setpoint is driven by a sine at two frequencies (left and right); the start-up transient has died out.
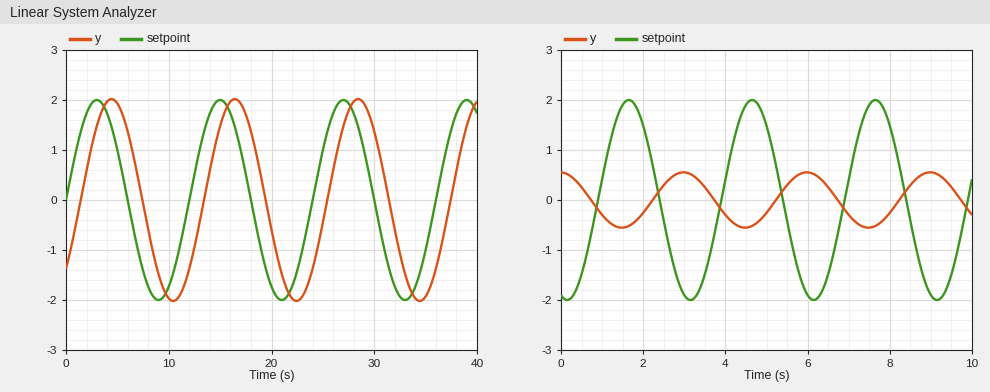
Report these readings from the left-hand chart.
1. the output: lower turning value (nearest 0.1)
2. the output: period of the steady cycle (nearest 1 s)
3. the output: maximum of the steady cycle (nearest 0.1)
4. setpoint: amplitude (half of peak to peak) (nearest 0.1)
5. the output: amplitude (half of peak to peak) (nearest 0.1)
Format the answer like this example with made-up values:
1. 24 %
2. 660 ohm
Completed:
1. -2.0
2. 12 s
3. 2.0
4. 2.0
5. 2.0
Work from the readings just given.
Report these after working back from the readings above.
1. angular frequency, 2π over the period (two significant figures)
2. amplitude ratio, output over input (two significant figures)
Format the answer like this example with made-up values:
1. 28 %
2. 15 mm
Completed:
1. 0.52 rad/s
2. 1.0
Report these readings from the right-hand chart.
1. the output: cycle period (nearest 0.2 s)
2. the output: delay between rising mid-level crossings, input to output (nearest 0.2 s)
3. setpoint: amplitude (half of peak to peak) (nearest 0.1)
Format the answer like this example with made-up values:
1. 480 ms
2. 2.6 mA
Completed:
1. 3.0 s
2. 1.4 s
3. 2.0
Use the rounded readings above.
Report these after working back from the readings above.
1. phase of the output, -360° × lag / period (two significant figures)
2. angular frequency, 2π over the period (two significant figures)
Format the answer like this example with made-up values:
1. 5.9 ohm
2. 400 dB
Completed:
1. -170°
2. 2.1 rad/s
